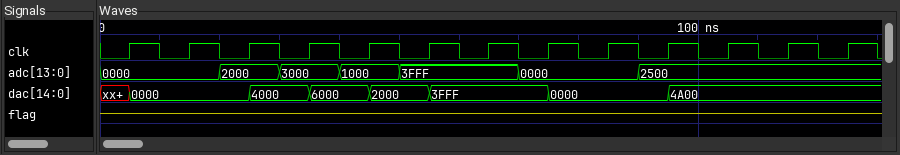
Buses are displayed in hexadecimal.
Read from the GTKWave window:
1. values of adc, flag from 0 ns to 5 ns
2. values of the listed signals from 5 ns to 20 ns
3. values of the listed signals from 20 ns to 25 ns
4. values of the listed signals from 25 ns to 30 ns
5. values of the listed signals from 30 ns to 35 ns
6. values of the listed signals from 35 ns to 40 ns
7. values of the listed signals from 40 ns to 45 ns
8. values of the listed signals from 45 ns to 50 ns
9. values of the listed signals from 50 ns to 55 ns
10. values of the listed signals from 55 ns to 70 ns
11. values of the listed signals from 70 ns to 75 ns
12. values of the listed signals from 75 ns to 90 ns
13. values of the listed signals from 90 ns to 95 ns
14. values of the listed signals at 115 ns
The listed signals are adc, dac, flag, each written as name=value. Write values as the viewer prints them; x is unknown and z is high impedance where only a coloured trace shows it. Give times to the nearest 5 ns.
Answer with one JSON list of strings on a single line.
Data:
["adc=0000, flag=z", "adc=0000, dac=0000, flag=z", "adc=2000, dac=0000, flag=z", "adc=2000, dac=4000, flag=z", "adc=3000, dac=4000, flag=z", "adc=3000, dac=6000, flag=z", "adc=1000, dac=6000, flag=z", "adc=1000, dac=2000, flag=z", "adc=3FFF, dac=2000, flag=z", "adc=3FFF, dac=3FFF, flag=z", "adc=0000, dac=3FFF, flag=z", "adc=0000, dac=0000, flag=z", "adc=2500, dac=0000, flag=z", "adc=2500, dac=4A00, flag=z"]
